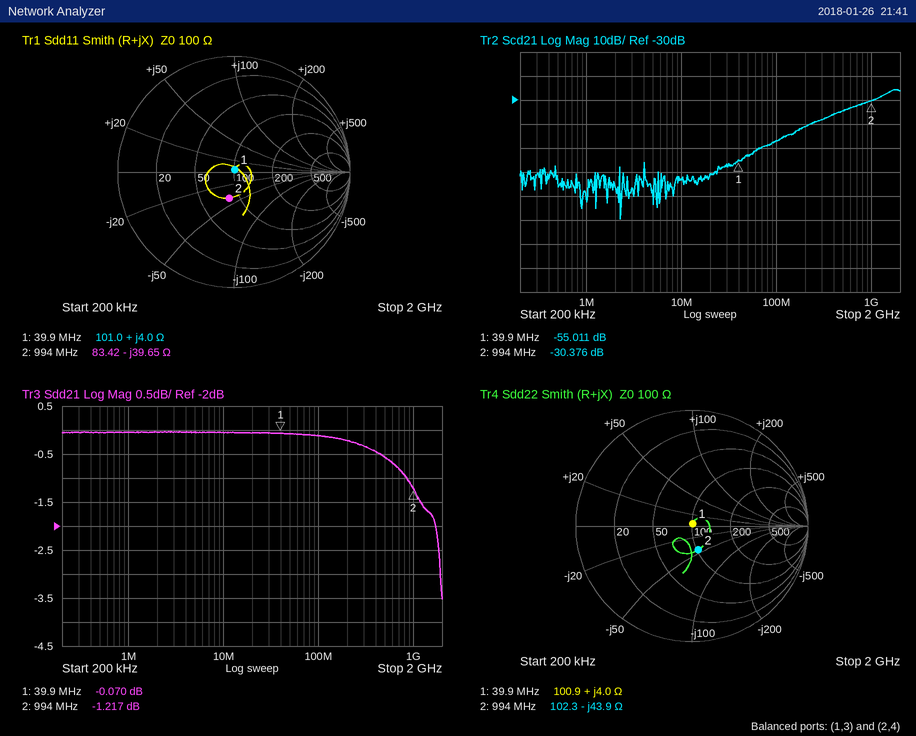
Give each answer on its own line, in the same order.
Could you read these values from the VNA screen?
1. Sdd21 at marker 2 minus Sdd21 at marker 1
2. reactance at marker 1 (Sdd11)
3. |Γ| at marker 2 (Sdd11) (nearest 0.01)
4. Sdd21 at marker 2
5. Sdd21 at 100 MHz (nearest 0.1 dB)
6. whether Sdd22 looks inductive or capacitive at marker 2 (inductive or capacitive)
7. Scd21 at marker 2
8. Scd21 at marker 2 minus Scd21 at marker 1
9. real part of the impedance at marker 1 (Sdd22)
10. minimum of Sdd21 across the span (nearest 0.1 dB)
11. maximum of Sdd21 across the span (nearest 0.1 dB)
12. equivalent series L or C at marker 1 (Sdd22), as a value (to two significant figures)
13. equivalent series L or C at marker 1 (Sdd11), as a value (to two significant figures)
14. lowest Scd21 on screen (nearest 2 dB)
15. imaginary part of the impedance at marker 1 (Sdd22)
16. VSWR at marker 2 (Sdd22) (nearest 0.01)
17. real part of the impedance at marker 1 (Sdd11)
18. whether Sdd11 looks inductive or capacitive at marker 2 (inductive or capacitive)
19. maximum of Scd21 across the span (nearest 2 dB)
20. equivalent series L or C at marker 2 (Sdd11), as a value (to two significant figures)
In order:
-1.147 dB
+4.0 Ω
0.23
-1.217 dB
-0.1 dB
capacitive
-30.376 dB
24.635 dB
100.9 Ω
-3.5 dB
0.0 dB
16 nH
16 nH
-80 dB
+4.0 Ω
1.54
101.0 Ω
capacitive
-26 dB
4.0 pF
